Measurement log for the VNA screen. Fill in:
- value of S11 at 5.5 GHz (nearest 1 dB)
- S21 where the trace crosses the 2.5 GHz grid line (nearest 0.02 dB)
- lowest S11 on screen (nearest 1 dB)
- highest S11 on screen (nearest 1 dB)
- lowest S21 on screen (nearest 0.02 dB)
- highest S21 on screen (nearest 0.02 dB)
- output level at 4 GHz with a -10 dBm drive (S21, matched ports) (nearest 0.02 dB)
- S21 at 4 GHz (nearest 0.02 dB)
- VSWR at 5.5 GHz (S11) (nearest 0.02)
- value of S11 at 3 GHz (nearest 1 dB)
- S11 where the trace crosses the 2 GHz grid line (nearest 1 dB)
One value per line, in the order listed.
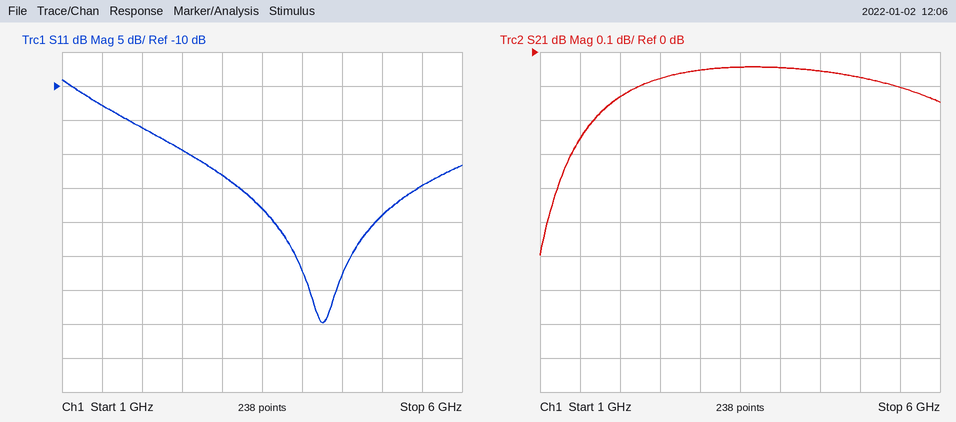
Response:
-25 dB
-0.08 dB
-45 dB
-9 dB
-0.60 dB
-0.04 dB
-10.04 dBm
-0.04 dB
1.12
-23 dB
-16 dB
